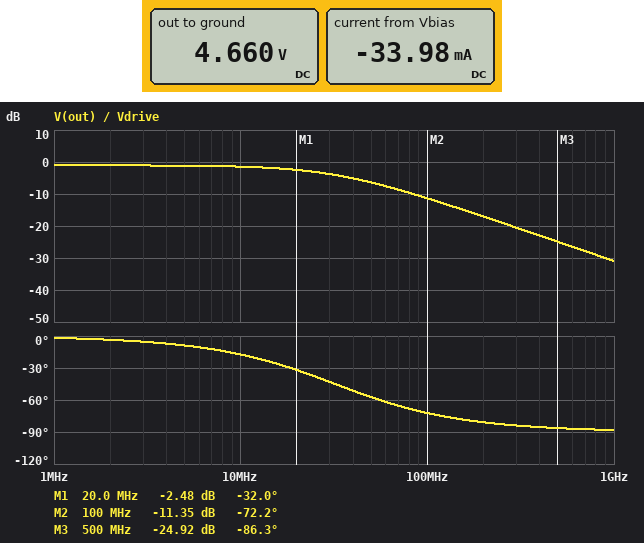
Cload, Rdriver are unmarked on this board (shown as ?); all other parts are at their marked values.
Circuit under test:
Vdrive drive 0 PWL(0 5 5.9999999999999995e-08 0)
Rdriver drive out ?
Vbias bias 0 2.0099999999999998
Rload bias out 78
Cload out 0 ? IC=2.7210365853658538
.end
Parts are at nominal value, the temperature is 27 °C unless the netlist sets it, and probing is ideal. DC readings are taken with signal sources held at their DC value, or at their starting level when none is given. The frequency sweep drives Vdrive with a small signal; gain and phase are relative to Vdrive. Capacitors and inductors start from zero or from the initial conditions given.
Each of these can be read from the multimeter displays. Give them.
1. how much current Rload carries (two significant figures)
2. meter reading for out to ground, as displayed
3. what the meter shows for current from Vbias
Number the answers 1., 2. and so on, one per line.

1. 34 mA
2. 4.660 V
3. -33.98 mA
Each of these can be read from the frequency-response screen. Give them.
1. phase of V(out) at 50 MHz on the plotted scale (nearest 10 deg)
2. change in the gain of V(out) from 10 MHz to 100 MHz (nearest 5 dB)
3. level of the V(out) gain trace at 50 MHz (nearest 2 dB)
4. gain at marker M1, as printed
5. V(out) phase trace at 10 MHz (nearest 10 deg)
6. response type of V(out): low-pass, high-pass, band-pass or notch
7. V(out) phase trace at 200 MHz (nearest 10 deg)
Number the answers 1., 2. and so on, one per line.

1. -60 deg
2. -10 dB
3. -6 dB
4. -2.48 dB
5. -20 deg
6. low-pass
7. -80 deg
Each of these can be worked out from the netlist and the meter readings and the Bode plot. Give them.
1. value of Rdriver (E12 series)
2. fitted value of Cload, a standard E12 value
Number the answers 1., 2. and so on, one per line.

1. 10 Ω
2. 560 pF
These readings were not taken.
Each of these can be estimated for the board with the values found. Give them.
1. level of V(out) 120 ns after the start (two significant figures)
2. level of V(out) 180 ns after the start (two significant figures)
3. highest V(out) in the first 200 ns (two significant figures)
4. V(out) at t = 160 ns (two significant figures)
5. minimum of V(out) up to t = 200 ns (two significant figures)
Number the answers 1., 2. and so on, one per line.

1. 230 mV
2. 230 mV
3. 4.0 V
4. 230 mV
5. 230 mV
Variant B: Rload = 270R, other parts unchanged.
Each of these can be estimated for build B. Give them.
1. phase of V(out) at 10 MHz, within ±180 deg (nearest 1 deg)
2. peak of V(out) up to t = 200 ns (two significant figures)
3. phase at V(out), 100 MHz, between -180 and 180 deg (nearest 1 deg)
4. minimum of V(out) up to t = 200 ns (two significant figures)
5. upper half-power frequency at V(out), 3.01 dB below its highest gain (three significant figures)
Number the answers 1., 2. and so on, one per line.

1. -19 deg
2. 4.1 V
3. -74 deg
4. 72 mV
5. 29.5 MHz
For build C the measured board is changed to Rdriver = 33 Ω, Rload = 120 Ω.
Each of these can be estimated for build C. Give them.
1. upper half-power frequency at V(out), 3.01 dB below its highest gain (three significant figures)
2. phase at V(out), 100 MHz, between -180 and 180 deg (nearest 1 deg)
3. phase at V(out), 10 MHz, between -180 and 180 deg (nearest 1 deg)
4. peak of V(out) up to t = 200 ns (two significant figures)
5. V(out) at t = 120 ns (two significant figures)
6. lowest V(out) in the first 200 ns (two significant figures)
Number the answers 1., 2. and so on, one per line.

1. 11.0 MHz
2. -84 deg
3. -42 deg
4. 3.4 V
5. 450 mV
6. 430 mV
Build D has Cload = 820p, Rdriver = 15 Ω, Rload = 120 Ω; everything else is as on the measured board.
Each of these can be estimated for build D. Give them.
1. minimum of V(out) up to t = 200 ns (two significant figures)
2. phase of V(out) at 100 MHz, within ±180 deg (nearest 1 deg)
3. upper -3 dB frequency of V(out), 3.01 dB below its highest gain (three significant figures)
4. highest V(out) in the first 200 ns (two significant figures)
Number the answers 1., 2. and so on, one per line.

1. 220 mV
2. -82 deg
3. 14.6 MHz
4. 3.7 V
